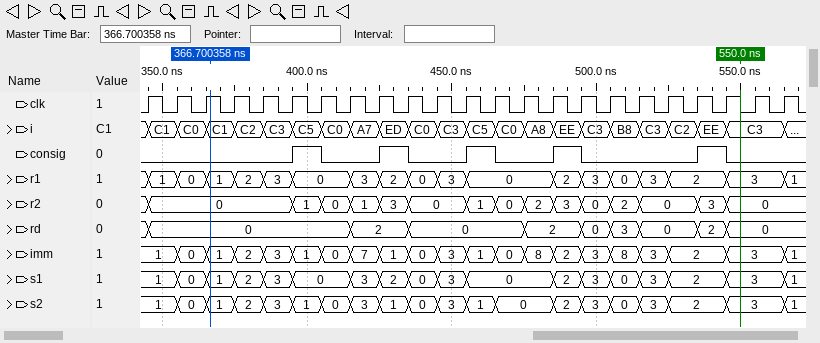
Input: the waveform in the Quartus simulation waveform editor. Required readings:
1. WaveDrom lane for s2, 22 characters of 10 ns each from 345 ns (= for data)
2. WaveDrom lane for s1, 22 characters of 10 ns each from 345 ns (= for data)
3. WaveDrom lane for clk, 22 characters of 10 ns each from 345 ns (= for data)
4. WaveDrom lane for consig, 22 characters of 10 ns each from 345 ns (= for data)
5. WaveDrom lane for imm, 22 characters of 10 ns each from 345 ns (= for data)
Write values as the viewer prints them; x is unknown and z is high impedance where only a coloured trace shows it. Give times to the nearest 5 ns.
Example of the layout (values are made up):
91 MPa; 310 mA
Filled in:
{name: 's2', wave: '=============.=====.=.', data: '1 0 1 2 3 1 0 3 1 0 3 1 0 2 3 0 3 2 3'}; {name: 's1', wave: '======.=====..=====.=.', data: '1 0 1 2 3 0 3 2 0 3 0 2 3 0 3 2 3'}; {name: 'clk', wave: 'p.....................'}; {name: 'consig', wave: '0....10.10.10.10...10.'}; {name: 'imm', wave: '===================.=.', data: '1 0 1 2 3 1 0 7 1 0 3 1 0 8 2 3 8 3 2 3'}
